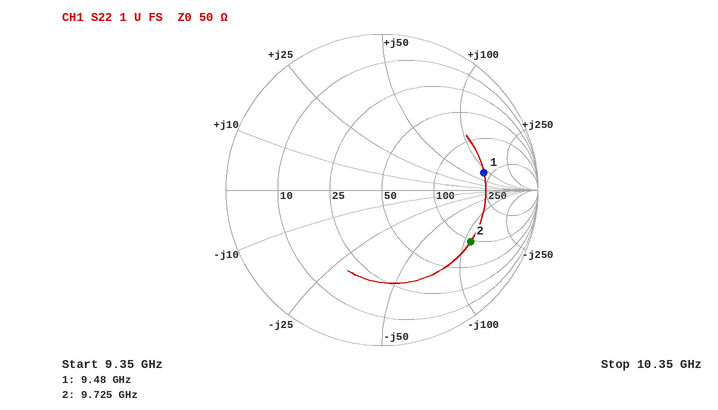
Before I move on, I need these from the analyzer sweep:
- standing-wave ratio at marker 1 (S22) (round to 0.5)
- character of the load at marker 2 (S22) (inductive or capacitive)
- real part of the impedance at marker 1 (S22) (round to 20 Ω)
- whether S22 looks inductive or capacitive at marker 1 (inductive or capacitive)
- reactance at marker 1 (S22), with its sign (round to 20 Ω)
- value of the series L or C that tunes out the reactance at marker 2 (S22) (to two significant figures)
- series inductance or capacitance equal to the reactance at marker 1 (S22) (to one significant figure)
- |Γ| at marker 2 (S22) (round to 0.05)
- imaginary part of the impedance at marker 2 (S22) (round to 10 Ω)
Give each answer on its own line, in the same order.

5.0
capacitive
220 Ω
inductive
+80 Ω
1.8 nH
1 nH
0.65
-110 Ω
